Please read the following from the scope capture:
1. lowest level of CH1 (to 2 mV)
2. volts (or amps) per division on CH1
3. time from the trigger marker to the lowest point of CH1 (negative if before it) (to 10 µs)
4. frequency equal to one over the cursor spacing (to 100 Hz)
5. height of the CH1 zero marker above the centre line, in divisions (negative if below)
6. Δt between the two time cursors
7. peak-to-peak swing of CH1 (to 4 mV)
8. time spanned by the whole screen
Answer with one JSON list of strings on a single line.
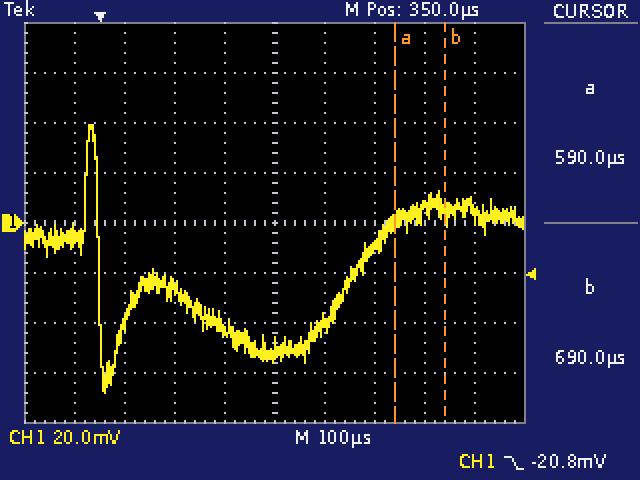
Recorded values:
["-68 mV", "20 mV", "+10 µs", "10.0 kHz", "0.0 div", "100 µs", "108 mV", "1 ms"]
